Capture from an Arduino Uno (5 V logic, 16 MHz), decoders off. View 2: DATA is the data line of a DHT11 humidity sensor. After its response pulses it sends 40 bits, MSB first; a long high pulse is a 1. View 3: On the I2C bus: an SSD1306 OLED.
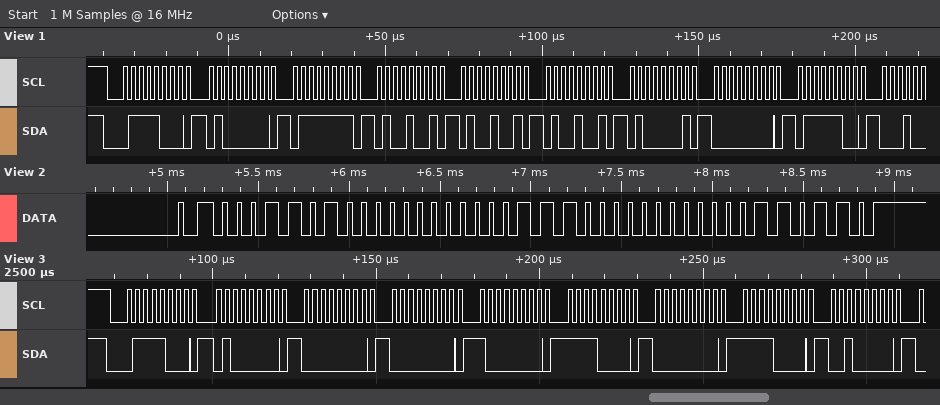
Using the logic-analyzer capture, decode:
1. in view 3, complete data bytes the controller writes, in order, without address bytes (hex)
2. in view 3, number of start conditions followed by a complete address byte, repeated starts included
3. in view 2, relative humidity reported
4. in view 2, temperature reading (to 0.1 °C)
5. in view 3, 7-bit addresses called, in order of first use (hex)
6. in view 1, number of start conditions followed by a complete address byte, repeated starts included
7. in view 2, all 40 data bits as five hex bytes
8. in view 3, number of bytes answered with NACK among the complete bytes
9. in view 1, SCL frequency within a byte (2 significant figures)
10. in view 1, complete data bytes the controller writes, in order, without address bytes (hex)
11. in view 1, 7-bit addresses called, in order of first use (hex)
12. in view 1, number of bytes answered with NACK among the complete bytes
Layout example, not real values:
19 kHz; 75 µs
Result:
40 00 00 80 F0 00 F0 20; 1; 26 %; 28.0 °C; 0x3C; 1; 1A 00 1C 00 36; 0; 400 kHz; 40 7F 49 49 49 41 00 7C; 0x3C; 0
